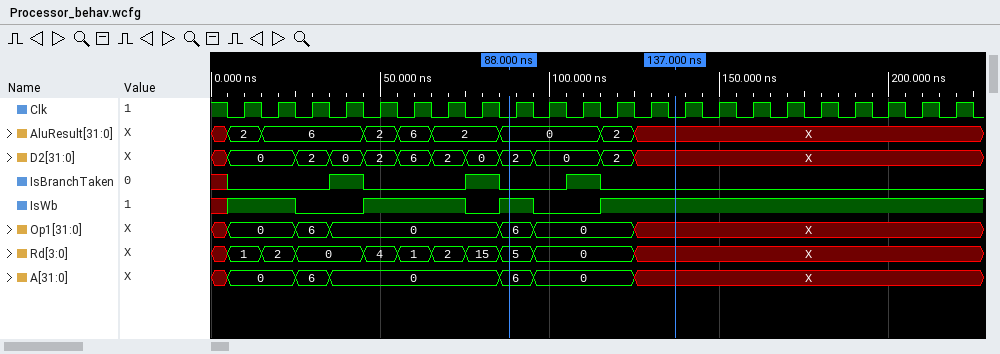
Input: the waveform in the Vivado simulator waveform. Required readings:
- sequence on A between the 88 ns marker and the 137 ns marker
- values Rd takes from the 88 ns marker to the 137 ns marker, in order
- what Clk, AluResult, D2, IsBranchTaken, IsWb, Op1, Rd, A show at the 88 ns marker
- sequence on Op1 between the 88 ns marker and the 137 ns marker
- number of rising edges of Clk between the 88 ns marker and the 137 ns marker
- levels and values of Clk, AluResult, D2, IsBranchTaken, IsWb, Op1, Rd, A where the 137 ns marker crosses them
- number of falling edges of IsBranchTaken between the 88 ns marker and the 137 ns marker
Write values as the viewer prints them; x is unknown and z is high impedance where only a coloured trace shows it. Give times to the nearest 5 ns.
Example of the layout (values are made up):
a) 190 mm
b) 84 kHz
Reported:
a) 6, 0, X
b) 5, 0, X
c) Clk=0, AluResult=0, D2=2, IsBranchTaken=0, IsWb=1, Op1=6, Rd=5, A=6
d) 6, 0, X
e) 5
f) Clk=0, AluResult=X, D2=X, IsBranchTaken=0, IsWb=1, Op1=X, Rd=X, A=X
g) 1
